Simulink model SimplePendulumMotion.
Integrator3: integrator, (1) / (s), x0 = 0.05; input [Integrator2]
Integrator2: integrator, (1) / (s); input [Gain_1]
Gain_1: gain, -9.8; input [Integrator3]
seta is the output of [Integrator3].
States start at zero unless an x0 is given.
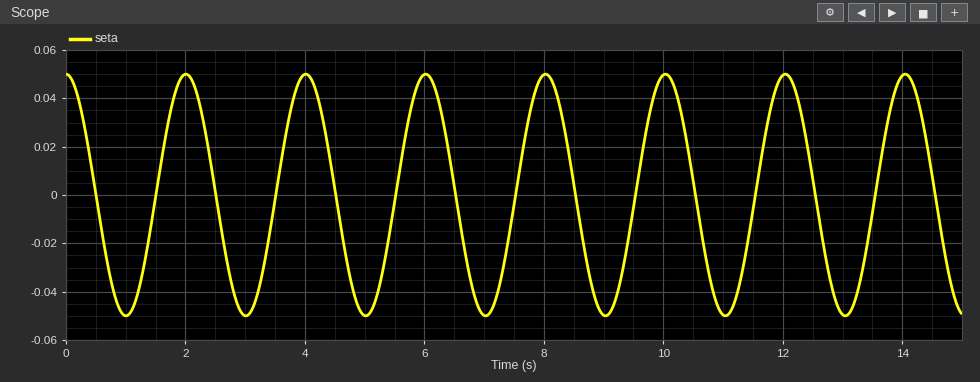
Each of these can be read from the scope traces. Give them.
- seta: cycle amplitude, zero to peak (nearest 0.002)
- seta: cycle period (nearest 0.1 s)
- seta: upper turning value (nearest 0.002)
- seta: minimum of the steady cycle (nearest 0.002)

0.050
2.0 s
0.050
-0.050
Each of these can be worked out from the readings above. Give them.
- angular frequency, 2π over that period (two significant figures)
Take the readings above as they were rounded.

3.1 rad/s
